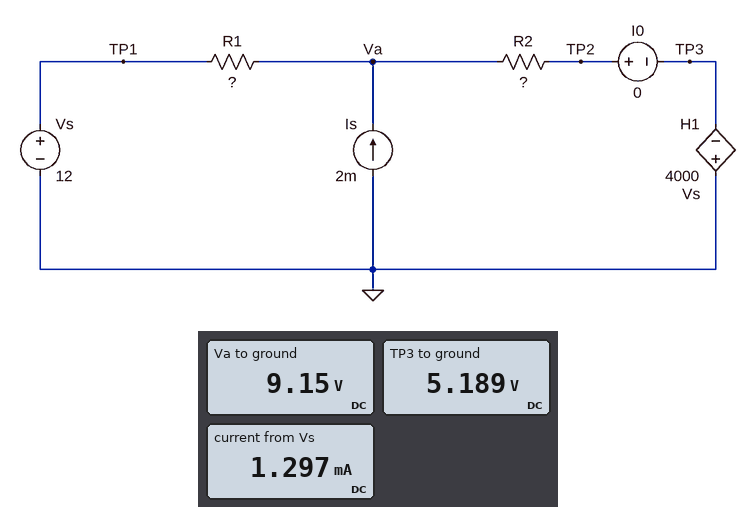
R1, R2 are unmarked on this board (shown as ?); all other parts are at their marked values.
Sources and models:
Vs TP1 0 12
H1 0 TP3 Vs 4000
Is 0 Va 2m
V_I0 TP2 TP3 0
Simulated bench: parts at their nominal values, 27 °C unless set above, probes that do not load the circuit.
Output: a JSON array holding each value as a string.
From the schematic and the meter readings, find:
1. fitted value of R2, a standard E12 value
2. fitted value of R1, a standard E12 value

["1.2 kΩ", "2.2 kΩ"]
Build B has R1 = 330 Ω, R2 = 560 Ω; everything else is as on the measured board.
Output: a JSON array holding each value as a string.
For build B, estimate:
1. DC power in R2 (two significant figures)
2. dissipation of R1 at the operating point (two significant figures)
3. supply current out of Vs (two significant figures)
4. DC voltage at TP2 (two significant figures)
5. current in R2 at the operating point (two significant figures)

["10 mW", "1.6 mW", "2.2 mA", "8.9 V", "4.2 mA"]
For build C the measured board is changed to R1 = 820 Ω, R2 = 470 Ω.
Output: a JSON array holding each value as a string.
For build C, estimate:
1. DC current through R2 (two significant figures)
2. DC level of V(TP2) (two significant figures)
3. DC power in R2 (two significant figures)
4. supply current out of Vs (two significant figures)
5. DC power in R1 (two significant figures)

["4.1 mA", "8.4 V", "7.9 mW", "2.1 mA", "3.6 mW"]
